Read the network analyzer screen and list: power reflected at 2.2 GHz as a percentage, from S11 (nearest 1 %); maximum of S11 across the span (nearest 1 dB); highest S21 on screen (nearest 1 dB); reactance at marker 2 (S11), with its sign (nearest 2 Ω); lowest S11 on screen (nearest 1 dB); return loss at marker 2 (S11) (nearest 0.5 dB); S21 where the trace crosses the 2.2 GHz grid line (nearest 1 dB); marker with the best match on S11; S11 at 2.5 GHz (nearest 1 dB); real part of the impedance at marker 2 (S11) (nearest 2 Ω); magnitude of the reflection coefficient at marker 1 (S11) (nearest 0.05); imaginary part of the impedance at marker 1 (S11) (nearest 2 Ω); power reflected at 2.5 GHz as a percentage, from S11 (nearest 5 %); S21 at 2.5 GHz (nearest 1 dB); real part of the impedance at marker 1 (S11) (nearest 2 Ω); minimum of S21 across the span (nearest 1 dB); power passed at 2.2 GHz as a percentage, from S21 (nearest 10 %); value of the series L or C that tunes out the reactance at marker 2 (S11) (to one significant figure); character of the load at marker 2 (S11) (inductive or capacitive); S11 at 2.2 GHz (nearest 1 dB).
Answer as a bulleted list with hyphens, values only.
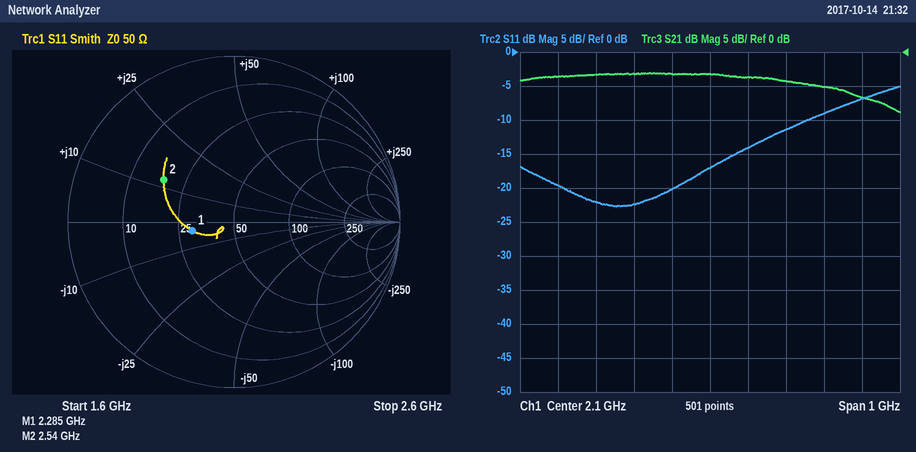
- 4 %
- -5 dB
- -3 dB
- +12 Ω
- -23 dB
- 6.0 dB
- -4 dB
- marker 1
- -7 dB
- 18 Ω
- 0.25
- -4 Ω
- 20 %
- -7 dB
- 30 Ω
- -9 dB
- 40 %
- 5 pF
- inductive
- -14 dB
